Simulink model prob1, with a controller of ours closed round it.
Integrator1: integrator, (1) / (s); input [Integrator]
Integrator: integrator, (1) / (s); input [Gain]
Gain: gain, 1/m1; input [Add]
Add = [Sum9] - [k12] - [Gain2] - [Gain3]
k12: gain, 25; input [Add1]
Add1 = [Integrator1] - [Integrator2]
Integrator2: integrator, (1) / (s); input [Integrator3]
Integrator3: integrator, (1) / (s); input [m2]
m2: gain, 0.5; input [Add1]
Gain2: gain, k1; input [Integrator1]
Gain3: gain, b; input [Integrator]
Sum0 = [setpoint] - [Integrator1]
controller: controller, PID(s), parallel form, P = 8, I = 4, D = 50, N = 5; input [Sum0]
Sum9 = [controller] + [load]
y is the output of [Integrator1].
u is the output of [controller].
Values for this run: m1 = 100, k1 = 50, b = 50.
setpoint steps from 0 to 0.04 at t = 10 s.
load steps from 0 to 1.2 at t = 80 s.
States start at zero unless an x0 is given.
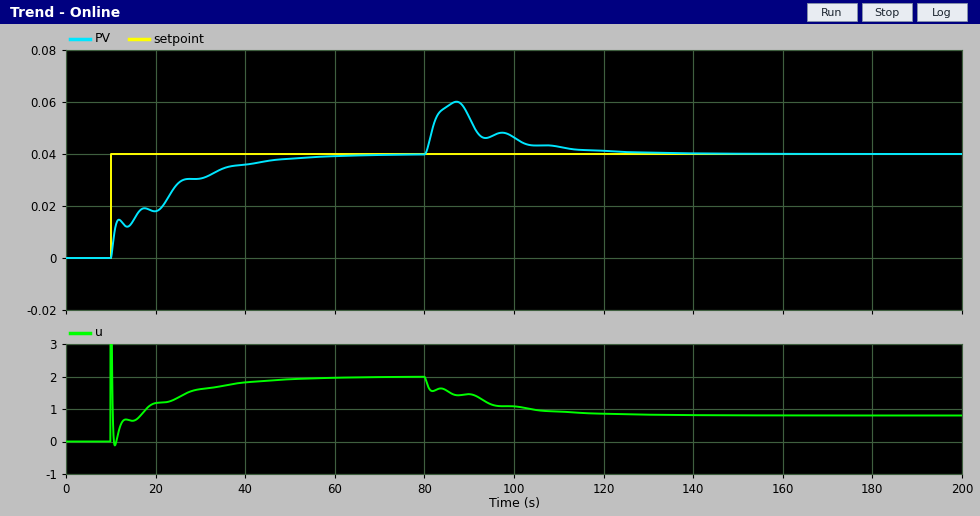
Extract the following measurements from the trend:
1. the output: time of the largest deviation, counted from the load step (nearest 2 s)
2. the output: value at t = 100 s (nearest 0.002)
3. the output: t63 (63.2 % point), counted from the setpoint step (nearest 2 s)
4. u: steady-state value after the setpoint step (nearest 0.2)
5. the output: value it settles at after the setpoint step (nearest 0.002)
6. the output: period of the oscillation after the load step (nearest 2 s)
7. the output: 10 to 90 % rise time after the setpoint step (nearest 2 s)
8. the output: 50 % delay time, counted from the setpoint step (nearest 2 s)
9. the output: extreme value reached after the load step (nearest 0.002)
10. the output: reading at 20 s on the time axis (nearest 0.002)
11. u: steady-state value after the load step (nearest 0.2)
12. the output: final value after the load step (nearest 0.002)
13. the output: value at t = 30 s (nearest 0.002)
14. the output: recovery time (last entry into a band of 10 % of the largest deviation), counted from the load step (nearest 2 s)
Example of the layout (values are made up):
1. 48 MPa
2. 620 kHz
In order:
1. 8 s
2. 0.046
3. 14 s
4. 2.0
5. 0.040
6. 10 s
7. 30 s
8. 12 s
9. 0.060
10. 0.018
11. 0.8
12. 0.040
13. 0.030
14. 32 s
